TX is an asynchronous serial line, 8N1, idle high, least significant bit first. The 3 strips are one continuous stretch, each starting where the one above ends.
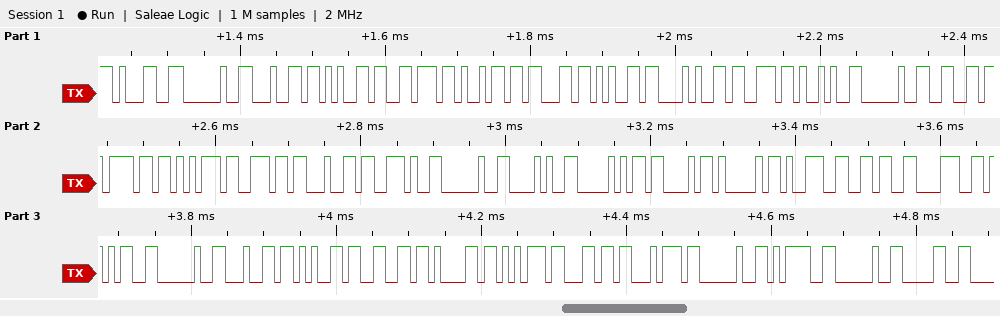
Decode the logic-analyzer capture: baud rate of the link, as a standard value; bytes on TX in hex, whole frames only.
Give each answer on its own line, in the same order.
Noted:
115200 baud
0x31 0x20 0x64 0x65 0x76 0x69 0x63 0x65 0x28 0x73 0x29 0x20 0x66 0x6F 0x75 0x6E 0x64 0x2E 0x20 0x28 0x50 0x43 0x41 0x39 0x36 0x38 0x35 0x20 0x64 0x65 0x66 0x61 0x75 0x6C 0x74 0x20 0x3D 0x20 0x30
